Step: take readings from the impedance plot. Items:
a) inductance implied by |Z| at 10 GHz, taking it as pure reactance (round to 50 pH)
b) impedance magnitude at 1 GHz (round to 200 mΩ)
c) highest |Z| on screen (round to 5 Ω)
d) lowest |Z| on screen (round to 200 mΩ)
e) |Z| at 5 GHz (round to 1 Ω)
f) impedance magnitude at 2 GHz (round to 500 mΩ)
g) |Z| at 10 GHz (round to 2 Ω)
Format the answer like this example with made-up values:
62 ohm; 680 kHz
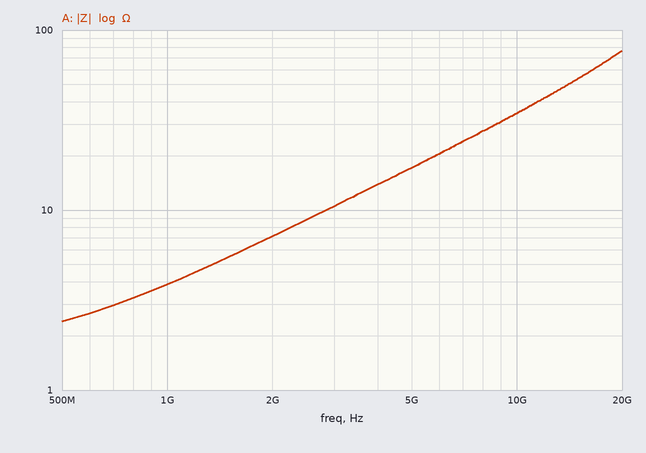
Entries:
550 pH; 3.8 Ω; 75 Ω; 2.4 Ω; 17 Ω; 7.0 Ω; 34 Ω
